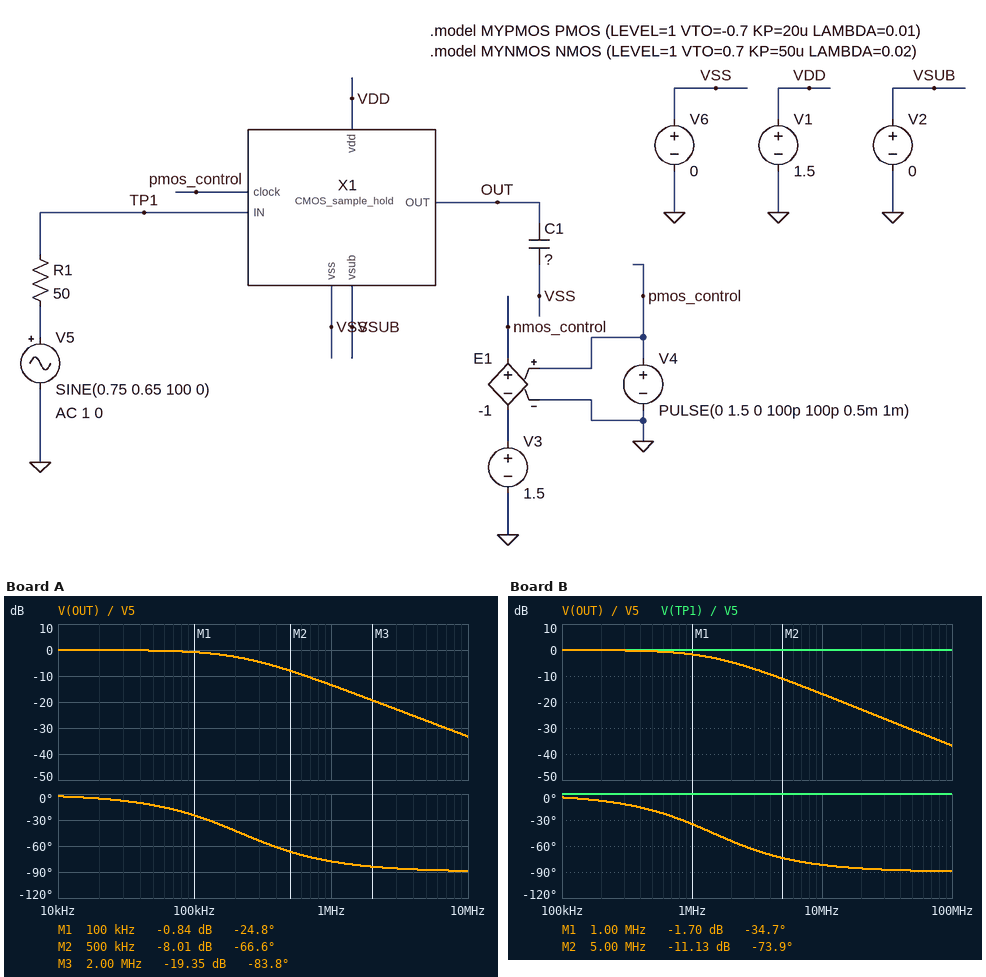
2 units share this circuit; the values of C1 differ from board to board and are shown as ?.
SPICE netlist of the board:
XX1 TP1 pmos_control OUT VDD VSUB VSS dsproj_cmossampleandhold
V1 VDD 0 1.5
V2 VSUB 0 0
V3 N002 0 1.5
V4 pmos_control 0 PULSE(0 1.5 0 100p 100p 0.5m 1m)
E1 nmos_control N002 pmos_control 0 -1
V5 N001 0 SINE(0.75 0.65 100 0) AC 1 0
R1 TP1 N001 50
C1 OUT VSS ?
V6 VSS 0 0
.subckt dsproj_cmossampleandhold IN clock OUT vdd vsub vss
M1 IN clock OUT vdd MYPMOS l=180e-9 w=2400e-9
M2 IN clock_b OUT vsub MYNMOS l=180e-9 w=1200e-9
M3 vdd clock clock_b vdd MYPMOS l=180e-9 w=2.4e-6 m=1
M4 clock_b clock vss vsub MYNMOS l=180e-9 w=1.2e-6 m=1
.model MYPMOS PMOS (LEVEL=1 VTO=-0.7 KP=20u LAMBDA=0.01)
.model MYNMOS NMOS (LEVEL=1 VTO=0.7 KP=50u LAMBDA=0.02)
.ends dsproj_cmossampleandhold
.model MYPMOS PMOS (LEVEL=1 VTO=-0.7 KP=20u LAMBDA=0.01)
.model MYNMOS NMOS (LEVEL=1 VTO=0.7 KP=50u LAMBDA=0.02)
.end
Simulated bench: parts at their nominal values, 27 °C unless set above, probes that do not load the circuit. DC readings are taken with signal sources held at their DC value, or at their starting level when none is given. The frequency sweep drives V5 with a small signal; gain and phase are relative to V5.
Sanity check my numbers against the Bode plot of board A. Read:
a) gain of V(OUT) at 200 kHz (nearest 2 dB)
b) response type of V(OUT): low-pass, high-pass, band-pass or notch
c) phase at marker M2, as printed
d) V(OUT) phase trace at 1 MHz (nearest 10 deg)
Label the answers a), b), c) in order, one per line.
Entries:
a) -2 dB
b) low-pass
c) -66.6 deg
d) -80 deg
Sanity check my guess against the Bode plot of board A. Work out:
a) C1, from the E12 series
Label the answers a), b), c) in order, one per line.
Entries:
a) 22 pF
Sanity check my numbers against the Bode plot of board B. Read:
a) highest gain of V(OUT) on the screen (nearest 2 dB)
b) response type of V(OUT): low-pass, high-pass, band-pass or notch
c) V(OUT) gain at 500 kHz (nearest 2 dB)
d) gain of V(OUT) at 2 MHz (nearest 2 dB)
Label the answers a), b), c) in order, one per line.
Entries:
a) 0 dB
b) low-pass
c) 0 dB
d) -4 dB
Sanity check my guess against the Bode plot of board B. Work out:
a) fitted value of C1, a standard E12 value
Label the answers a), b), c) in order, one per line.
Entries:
a) 3.3 pF
